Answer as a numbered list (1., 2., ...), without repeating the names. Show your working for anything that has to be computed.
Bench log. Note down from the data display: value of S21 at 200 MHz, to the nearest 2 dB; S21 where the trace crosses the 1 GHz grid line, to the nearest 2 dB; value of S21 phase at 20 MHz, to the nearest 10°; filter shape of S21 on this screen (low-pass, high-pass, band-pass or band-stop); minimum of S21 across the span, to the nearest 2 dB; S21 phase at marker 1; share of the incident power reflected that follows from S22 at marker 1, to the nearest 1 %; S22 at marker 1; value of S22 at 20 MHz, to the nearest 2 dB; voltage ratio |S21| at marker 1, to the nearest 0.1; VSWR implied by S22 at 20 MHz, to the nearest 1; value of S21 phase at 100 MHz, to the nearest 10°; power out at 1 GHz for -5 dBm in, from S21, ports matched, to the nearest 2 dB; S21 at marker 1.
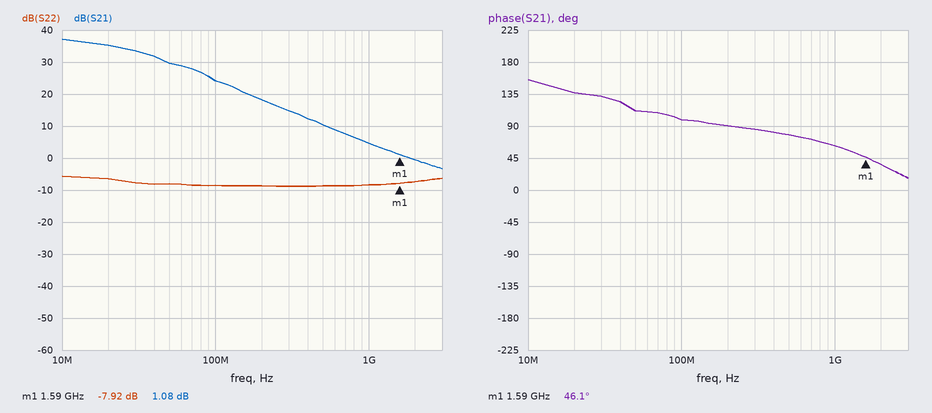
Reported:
1. 18 dB
2. 4 dB
3. 140°
4. low-pass
5. -4 dB
6. 46.1°
7. 10^(-7.92/10) ≈ 16 %
8. -7.92 dB
9. -6 dB
10. 10^(1.08/20) ≈ 1.1
11. |Γ| = 10^(-6/20) = 0.5012; VSWR = (1 + 0.5012)/(1 − 0.5012) ≈ 3
12. 100°
13. -5 dBm + (4 dB) = 0 dBm
14. 1.08 dB
